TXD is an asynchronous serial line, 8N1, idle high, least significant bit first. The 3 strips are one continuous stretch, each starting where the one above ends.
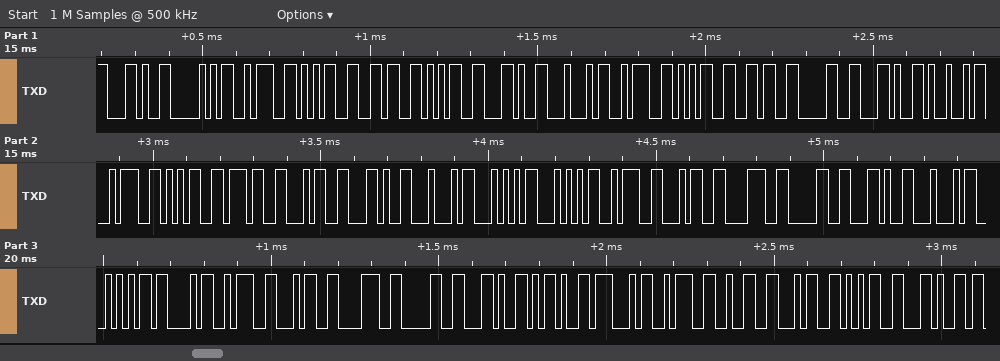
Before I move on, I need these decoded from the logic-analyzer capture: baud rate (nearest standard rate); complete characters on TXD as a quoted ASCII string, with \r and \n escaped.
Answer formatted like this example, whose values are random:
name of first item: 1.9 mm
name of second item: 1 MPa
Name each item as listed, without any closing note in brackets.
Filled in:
baud rate: 57600 baud
complete characters on TXD as a quoted ASCII string, with \r and \n escaped: ",P:565,D:560,I:574,DTT:480,DTC:480,-G:245,"
